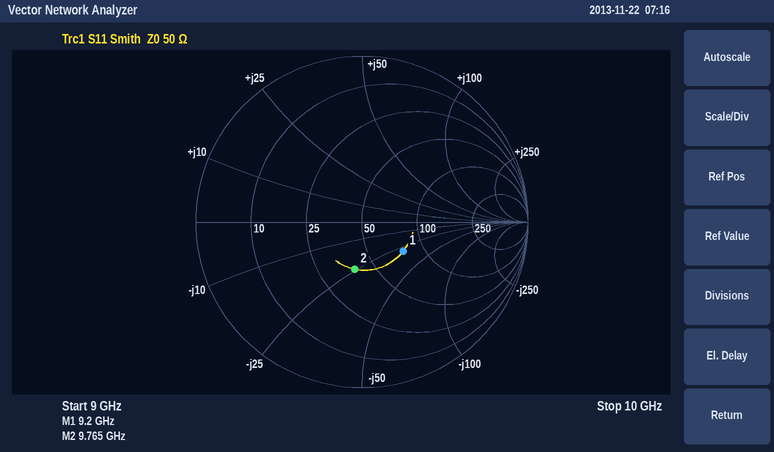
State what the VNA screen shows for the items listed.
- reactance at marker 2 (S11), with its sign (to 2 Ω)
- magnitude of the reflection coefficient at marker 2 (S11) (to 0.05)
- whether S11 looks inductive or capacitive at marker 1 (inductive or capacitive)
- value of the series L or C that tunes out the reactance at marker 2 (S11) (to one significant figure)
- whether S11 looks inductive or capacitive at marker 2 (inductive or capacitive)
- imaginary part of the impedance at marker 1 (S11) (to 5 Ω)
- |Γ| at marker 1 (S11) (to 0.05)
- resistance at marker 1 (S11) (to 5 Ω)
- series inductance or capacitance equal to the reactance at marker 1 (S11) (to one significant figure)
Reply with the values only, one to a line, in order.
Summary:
-24 Ω
0.30
capacitive
400 pH
capacitive
-30 Ω
0.30
75 Ω
600 fF
